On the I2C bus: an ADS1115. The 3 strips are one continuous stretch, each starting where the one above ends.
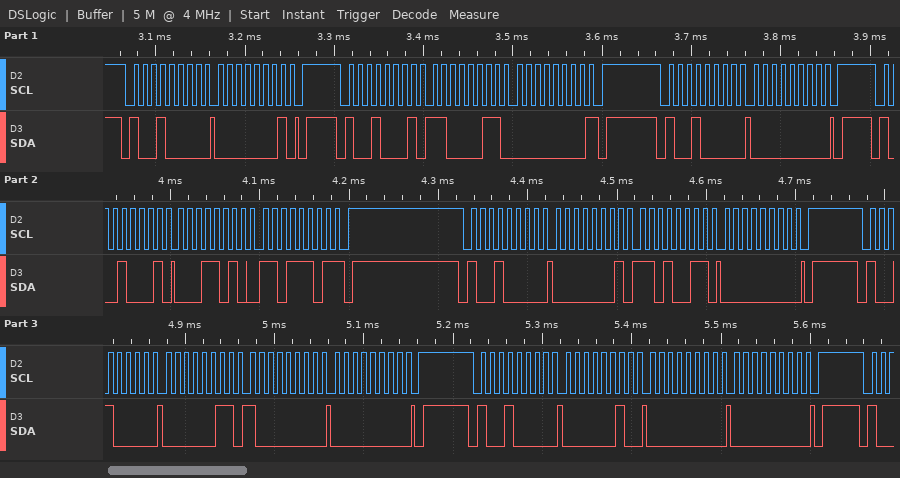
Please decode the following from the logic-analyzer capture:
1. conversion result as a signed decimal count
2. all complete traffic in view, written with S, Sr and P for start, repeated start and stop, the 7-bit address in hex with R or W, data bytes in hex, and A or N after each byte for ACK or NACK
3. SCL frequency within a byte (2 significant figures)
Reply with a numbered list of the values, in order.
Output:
1. 6877
2. S 48W A 01 A P S 48R A C3 A 00 N P S 48W A 00 A P S 48R A 1A A DD N P S 48W A 01 A D3 A 00 A P S 48W A 03 A 80 A 00 A P S 48W A 02 A 00 A 00 A P
3. 100 kHz
